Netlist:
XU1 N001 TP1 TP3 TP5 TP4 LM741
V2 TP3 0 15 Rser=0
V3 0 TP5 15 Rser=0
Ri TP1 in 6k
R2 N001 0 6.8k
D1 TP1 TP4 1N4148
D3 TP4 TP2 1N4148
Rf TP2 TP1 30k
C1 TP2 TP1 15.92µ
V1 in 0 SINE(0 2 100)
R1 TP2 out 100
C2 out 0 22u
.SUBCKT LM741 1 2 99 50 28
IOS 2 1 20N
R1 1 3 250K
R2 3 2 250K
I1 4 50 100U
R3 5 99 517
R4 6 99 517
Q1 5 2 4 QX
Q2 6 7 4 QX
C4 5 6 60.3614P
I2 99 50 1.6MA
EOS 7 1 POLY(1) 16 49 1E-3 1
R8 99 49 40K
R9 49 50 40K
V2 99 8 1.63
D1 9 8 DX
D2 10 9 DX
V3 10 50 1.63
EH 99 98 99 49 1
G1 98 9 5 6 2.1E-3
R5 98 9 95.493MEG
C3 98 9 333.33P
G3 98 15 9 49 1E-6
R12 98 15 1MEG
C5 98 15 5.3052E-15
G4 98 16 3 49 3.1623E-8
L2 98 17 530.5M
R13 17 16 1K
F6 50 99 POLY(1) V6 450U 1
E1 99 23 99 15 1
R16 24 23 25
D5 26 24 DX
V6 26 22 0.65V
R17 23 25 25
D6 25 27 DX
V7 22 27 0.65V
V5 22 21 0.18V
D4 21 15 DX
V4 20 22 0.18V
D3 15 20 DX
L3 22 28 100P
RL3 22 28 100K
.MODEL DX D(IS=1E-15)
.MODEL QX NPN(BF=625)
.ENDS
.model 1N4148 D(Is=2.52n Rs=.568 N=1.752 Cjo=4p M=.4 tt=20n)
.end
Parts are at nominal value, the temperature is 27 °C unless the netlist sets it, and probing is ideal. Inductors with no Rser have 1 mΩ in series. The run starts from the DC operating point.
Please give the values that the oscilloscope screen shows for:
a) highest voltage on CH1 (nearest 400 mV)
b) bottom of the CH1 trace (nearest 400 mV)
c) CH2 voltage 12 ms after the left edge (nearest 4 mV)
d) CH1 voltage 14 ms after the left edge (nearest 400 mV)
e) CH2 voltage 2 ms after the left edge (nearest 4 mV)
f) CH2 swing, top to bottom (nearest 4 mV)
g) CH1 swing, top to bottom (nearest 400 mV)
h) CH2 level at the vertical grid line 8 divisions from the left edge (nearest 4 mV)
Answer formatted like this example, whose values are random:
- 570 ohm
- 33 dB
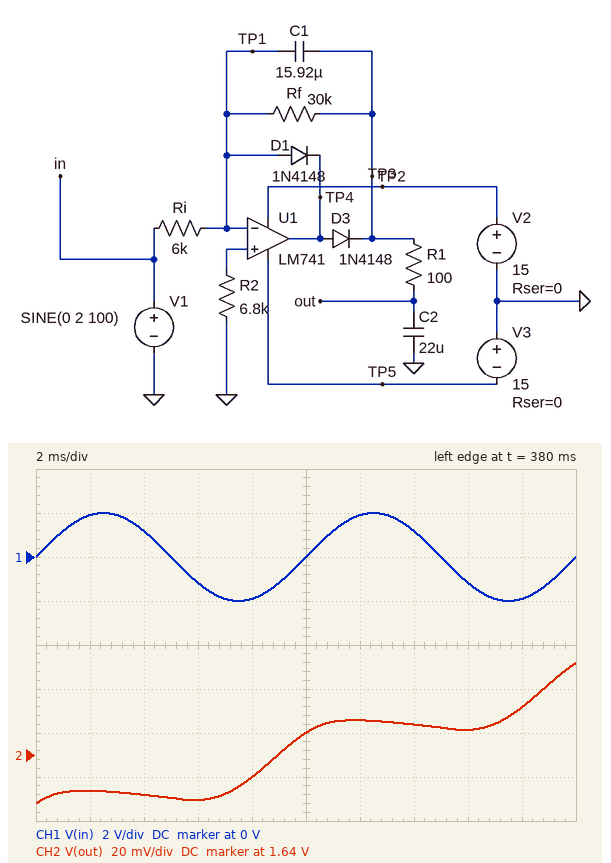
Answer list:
- 2.0 V
- -2.0 V
- 1.656 V
- 1.2 V
- 1.624 V
- 64 mV
- 4.0 V
- 1.652 V
